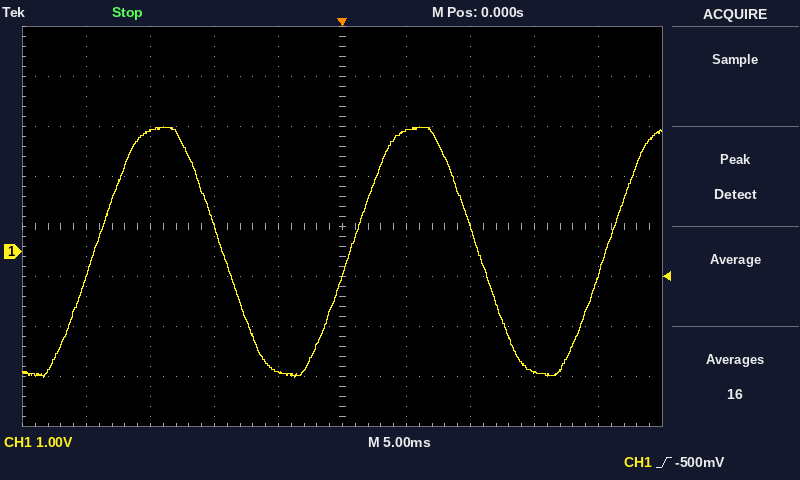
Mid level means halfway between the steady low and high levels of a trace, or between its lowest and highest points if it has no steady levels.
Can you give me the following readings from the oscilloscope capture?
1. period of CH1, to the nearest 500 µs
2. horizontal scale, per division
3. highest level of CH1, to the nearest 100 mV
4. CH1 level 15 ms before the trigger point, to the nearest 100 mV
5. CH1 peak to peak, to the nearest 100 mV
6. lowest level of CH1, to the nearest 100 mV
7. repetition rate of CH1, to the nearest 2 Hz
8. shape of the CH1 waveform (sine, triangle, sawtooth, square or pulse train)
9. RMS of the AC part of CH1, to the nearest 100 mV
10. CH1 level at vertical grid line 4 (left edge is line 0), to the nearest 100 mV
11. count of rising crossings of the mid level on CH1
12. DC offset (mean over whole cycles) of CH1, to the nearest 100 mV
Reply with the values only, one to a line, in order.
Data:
20.0 ms
5 ms
2.5 V
2.4 V
5.0 V
-2.5 V
50 Hz
sine
1.8 V
-2.4 V
3
0.0 V
